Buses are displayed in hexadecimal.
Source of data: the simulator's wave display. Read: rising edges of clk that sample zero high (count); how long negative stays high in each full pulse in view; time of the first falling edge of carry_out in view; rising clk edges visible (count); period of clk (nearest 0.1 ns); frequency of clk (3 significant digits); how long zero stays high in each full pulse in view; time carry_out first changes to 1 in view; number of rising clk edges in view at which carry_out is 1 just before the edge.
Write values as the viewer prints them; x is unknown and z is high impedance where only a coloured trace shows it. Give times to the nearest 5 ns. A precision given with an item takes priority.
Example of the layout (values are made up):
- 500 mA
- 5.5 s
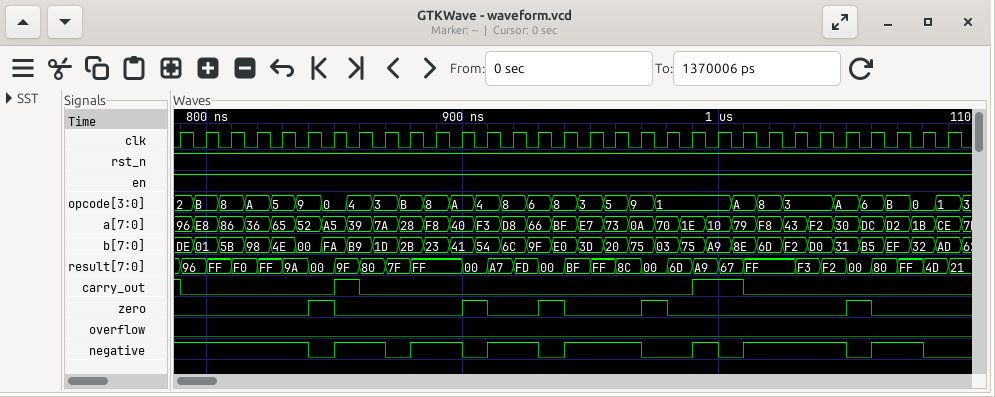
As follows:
- 5
- 20 ns, 20 ns, 20 ns, 30 ns, 10 ns, 40 ns, 20 ns
- 790 ns
- 31
- 10 ns
- 100 MHz
- 10 ns, 10 ns, 10 ns, 10 ns, 10 ns
- 850 ns
- 4
